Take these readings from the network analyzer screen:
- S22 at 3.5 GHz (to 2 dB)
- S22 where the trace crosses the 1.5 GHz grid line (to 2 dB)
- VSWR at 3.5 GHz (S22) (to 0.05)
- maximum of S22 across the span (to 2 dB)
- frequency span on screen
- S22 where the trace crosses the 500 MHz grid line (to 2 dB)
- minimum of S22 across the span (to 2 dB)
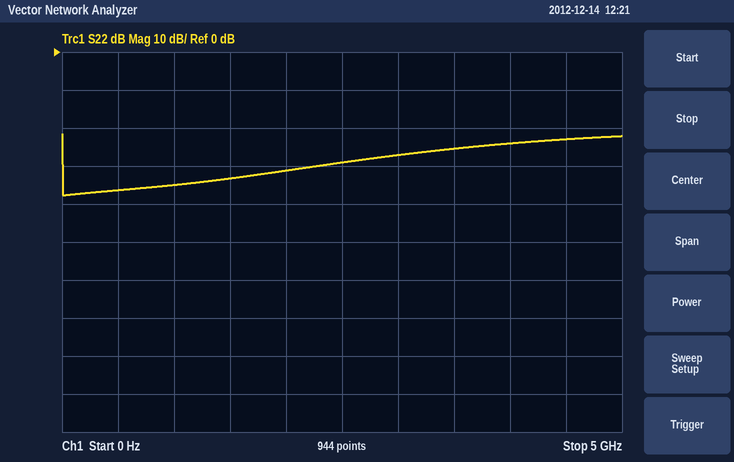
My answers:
-26 dB
-34 dB
1.10
-22 dB
5 GHz
-36 dB
-38 dB
